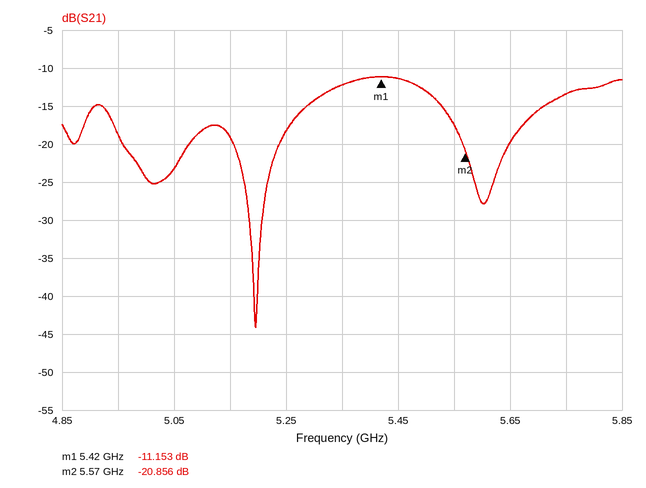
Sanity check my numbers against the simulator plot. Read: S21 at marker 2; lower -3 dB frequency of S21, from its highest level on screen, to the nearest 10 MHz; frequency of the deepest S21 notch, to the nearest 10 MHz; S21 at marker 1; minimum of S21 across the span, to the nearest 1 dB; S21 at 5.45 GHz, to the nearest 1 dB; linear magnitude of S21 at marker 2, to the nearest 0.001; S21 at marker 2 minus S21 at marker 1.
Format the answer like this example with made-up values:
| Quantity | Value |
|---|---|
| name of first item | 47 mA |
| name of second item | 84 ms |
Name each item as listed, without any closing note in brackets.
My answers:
| Quantity | Value |
|---|---|
| S21 at marker 2 | -20.856 dB |
| lower -3 dB frequency of S21, from its highest level on screen, to the nearest 10 MHz | 5.30 GHz |
| frequency of the deepest S21 notch, to the nearest 10 MHz | 5.20 GHz |
| S21 at marker 1 | -11.153 dB |
| minimum of S21 across the span, to the nearest 1 dB | -44 dB |
| S21 at 5.45 GHz, to the nearest 1 dB | -11 dB |
| linear magnitude of S21 at marker 2, to the nearest 0.001 | 0.091 |
| S21 at marker 2 minus S21 at marker 1 | -9.703 dB |
